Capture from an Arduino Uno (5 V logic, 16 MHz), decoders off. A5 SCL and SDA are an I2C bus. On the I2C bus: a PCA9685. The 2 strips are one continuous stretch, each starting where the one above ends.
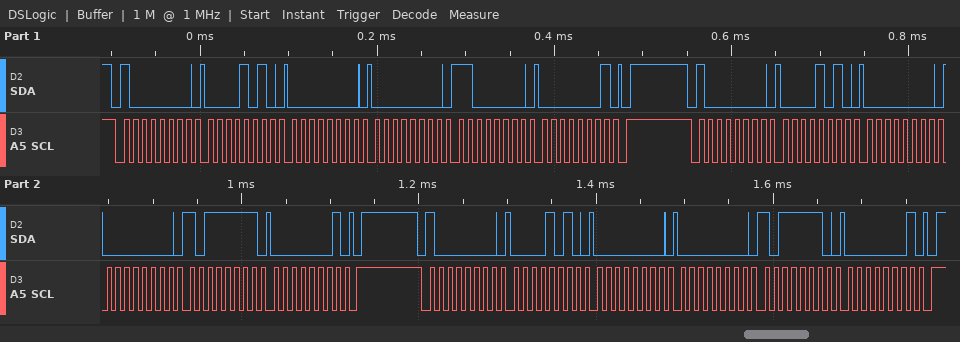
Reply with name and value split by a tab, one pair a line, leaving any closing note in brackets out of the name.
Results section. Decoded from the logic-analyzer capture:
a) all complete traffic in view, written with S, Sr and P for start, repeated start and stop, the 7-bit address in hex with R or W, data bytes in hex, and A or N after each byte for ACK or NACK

all complete traffic in view, written with S, Sr and P for start, repeated start and stop, the 7-bit address in hex with R or W, data bytes in hex, and A or N after each byte for ACK or NACK	S 40W A 0A A 00 A 00 A C0 A 01 A P S 40W A 0A A 00 A 00 A BF A 01 A P S 40W A 0A A 00 A 00 A BE A 01 A P
